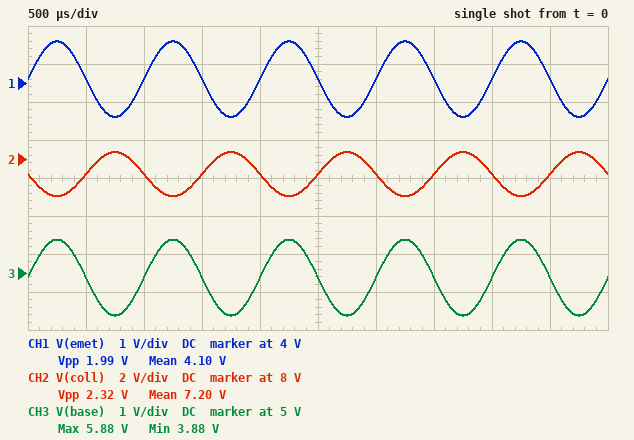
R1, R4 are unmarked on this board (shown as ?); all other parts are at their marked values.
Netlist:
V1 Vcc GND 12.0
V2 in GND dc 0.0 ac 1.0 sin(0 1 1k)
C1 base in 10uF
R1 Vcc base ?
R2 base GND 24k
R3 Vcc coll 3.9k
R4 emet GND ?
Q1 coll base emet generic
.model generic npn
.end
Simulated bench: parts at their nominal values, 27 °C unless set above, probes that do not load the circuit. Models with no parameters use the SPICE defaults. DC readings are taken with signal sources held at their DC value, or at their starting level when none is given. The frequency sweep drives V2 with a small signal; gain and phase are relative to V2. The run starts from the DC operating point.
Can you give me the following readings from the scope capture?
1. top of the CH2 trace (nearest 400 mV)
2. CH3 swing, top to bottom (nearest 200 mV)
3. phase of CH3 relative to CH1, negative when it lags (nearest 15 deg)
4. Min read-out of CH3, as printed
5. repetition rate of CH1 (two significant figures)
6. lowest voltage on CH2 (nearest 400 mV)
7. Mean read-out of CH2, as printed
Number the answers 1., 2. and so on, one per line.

1. 8.4 V
2. 2.0 V
3. 0 deg
4. 3.88 V
5. 1.0 kHz
6. 6.0 V
7. 7.20 V
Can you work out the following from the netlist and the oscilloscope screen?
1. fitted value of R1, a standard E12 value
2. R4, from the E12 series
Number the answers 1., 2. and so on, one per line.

1. 33 kΩ
2. 3.3 kΩ
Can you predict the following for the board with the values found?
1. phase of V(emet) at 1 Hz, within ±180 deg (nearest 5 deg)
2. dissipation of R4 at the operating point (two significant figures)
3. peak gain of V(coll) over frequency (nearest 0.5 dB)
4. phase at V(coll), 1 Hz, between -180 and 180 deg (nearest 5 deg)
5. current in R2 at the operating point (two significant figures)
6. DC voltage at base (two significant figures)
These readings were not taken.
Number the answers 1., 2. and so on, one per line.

1. 50 deg
2. 5.1 mW
3. 1.5 dB
4. -130 deg
5. 200 µA
6. 4.9 V
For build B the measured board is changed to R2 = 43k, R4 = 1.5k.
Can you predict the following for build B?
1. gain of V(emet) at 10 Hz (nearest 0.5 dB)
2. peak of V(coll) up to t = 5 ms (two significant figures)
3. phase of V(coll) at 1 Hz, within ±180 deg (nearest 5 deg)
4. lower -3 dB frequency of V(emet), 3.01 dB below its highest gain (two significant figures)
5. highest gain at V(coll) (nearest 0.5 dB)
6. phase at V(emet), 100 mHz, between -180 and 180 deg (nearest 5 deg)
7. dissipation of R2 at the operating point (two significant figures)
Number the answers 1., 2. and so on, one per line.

1. -5.0 dB
2. 5.9 V
3. 85 deg
4. 15 Hz
5. -2.0 dB
6. 90 deg
7. 420 µW
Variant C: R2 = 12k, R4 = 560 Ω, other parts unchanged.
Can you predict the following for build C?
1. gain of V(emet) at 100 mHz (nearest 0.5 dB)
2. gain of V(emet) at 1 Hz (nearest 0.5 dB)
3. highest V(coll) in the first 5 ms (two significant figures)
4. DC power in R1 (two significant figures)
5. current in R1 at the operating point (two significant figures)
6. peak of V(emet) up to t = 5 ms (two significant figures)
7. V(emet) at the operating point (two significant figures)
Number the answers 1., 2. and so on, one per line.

1. -50.0 dB
2. -30.0 dB
3. 9.6 V
4. 2.8 mW
5. 290 µA
6. 2.5 V
7. 1.5 V
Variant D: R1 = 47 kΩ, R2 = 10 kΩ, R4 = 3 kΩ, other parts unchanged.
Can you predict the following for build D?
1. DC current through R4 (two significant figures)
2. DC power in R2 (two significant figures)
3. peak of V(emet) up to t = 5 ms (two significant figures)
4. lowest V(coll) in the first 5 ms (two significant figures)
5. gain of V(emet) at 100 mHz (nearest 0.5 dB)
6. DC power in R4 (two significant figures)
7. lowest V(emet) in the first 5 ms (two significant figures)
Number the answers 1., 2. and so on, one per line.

1. 440 µA
2. 430 µW
3. 2.3 V
4. 9.0 V
5. -26.0 dB
6. 580 µW
7. 350 mV
